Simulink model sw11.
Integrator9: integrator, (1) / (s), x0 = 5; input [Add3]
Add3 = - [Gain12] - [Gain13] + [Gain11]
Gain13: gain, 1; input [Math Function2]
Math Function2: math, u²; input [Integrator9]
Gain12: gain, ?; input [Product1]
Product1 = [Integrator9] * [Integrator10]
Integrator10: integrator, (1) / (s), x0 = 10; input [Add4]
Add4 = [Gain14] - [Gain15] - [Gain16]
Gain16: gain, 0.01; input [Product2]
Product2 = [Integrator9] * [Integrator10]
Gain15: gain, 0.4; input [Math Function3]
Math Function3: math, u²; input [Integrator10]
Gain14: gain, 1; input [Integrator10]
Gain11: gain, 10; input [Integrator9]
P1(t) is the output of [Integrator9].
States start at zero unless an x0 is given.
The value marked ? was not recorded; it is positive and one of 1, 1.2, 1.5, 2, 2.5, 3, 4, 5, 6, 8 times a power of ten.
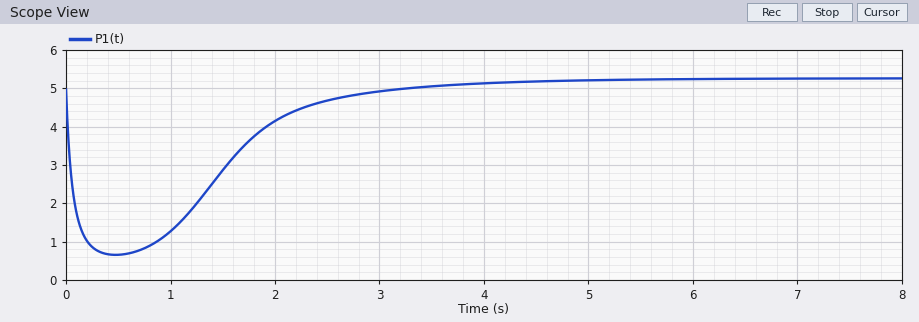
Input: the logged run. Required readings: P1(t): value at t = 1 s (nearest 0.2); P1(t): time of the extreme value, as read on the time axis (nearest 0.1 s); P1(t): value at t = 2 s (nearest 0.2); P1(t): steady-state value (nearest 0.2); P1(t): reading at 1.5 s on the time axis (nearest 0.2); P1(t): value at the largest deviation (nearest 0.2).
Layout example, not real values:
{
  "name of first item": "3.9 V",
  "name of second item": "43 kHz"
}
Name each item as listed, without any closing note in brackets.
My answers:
{
  "P1(t): value at t = 1 s": "1.2",
  "P1(t): time of the extreme value, as read on the time axis": "0.5 s",
  "P1(t): value at t = 2 s": "4.2",
  "P1(t): steady-state value": "5.2",
  "P1(t): reading at 1.5 s on the time axis": "2.8",
  "P1(t): value at the largest deviation": "0.6"
}
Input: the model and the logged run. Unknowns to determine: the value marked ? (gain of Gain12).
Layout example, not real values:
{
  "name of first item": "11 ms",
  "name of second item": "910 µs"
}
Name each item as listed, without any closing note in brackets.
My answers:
{
  "the value marked ?": "2"
}
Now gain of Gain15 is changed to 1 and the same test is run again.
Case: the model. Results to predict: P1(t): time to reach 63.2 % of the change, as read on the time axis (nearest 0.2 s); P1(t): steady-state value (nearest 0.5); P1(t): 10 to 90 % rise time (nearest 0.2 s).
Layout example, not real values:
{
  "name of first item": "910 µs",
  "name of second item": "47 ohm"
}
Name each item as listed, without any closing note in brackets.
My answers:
{
  "P1(t): time to reach 63.2 % of the change, as read on the time axis": "1.2 s",
  "P1(t): steady-state value": "8.0",
  "P1(t): 10 to 90 % rise time": "1.4 s"
}
